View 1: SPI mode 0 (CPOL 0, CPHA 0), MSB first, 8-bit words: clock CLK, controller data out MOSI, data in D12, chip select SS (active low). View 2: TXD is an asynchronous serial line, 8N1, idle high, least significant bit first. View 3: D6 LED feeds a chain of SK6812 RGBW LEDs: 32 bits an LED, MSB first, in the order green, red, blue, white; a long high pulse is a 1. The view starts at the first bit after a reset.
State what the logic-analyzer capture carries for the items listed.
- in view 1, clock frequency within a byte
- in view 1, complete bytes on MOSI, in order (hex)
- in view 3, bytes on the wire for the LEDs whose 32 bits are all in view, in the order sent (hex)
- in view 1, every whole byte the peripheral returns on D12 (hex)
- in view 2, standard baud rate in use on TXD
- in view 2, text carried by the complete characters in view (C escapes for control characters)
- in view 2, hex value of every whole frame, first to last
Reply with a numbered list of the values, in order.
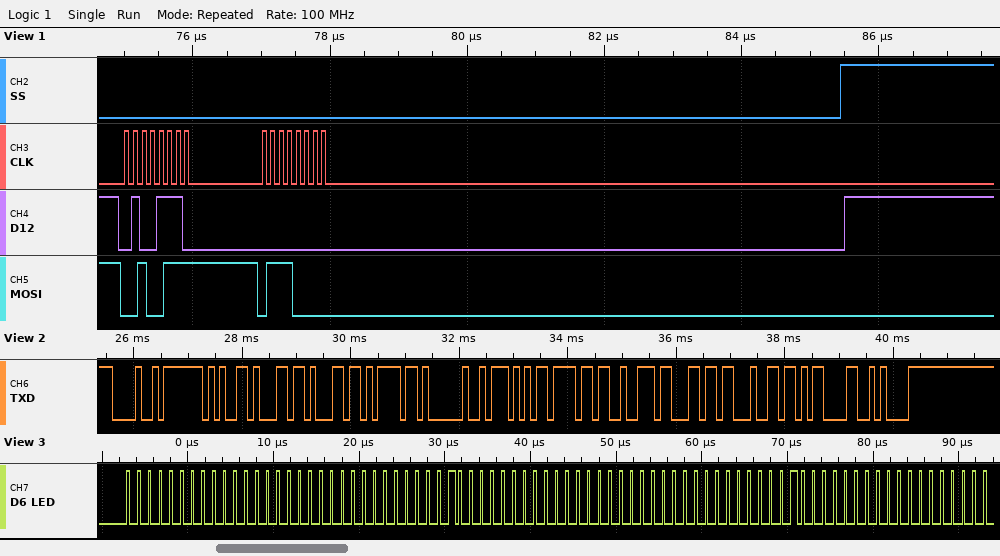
1. 8 MHz
2. 27 70
3. 00 00 00 02 00 00 00 02
4. 4E 00
5. 9600 baud
6. "Hello World\r\n"
7. 48 65 6C 6C 6F 20 57 6F 72 6C 64 0D 0A
